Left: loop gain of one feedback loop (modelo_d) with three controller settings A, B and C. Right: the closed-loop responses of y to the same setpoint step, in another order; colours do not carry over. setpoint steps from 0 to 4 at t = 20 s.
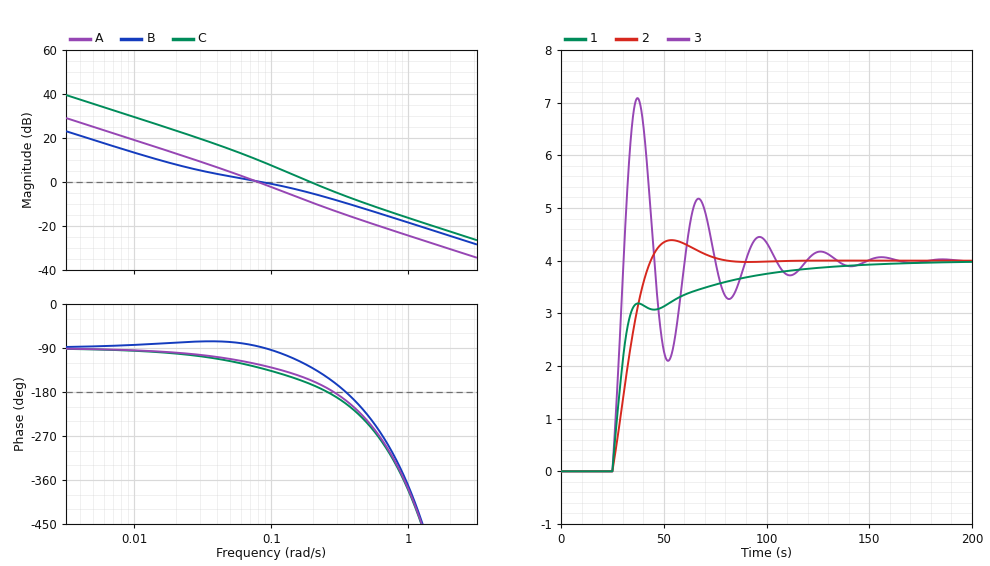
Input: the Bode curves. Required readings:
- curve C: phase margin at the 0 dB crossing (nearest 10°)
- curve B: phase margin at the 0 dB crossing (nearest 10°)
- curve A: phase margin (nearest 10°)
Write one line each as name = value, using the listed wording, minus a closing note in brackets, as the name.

curve C: phase margin at the 0 dB crossing = 20°
curve B: phase margin at the 0 dB crossing = 90°
curve A: phase margin = 60°
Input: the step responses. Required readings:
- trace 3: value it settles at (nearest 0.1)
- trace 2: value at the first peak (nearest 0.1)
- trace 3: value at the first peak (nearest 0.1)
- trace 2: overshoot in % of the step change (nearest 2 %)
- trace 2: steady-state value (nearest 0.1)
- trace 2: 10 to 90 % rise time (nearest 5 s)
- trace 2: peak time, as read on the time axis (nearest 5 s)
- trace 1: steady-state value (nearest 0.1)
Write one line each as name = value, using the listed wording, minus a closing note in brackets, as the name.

trace 3: value it settles at = 4.0
trace 2: value at the first peak = 4.4
trace 3: value at the first peak = 7.1
trace 2: overshoot in % of the step change = 10 %
trace 2: steady-state value = 4.0
trace 2: 10 to 90 % rise time = 15 s
trace 2: peak time, as read on the time axis = 55 s
trace 1: steady-state value = 4.0
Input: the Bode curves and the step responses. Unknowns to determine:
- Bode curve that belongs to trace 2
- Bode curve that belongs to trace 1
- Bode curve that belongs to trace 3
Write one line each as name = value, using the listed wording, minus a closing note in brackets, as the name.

Bode curve that belongs to trace 2 = A
Bode curve that belongs to trace 1 = B
Bode curve that belongs to trace 3 = C
